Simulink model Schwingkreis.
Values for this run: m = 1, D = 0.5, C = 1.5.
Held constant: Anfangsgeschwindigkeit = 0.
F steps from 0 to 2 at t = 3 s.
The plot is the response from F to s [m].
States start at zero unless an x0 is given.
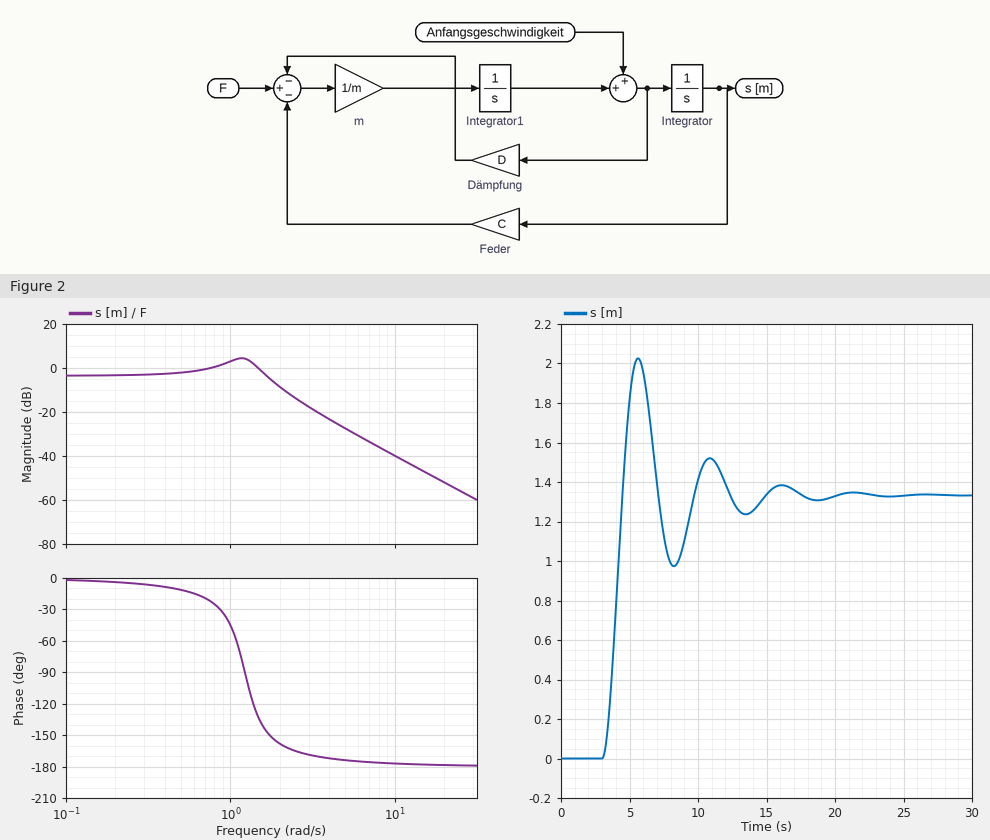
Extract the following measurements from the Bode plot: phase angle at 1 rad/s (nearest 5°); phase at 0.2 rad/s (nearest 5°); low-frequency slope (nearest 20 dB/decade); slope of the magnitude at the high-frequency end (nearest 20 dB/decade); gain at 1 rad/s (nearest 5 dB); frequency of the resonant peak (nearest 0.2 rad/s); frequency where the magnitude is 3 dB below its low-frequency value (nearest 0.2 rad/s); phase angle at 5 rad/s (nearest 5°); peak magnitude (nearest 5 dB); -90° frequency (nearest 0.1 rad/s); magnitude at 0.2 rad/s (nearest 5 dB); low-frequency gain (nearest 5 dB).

-45°
-5°
0 dB/decade
-40 dB/decade
5 dB
1.2 rad/s
1.8 rad/s
-175°
5 dB
1.2 rad/s
-5 dB
-5 dB
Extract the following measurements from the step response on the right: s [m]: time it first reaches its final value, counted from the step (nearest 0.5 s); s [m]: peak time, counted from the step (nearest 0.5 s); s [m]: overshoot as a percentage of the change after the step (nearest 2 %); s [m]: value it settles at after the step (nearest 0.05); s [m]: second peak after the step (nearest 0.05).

1.5 s
2.5 s
52 %
1.35
1.50
